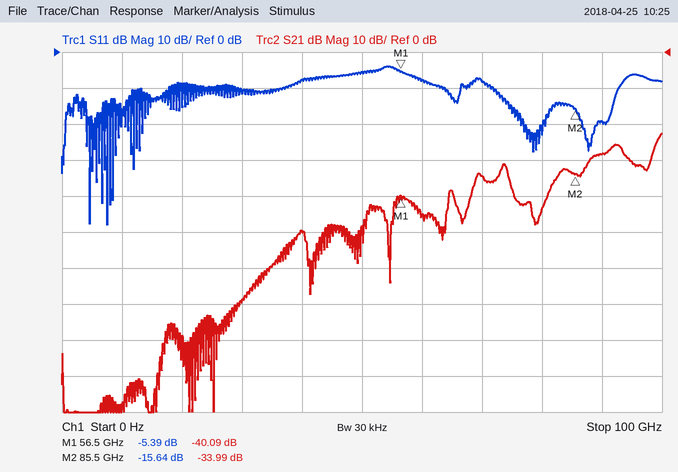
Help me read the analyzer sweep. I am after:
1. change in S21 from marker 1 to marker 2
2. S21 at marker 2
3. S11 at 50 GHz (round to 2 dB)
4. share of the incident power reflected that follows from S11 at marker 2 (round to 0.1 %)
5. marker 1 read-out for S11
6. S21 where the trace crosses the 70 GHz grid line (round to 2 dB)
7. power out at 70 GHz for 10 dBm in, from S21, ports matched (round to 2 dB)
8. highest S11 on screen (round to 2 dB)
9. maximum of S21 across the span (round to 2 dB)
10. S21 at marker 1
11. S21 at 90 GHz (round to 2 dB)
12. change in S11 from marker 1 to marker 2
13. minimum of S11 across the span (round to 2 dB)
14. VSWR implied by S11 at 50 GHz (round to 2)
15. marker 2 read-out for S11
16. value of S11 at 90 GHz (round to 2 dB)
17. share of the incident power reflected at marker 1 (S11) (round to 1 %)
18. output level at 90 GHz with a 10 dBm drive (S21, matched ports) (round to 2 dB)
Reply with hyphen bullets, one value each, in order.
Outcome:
- 6.10 dB
- -33.99 dB
- -6 dB
- 2.7 %
- -5.39 dB
- -34 dB
- -24 dBm
- -4 dB
- -22 dB
- -40.09 dB
- -28 dB
- -10.25 dB
- -48 dB
- 4
- -15.64 dB
- -20 dB
- 29 %
- -18 dBm
